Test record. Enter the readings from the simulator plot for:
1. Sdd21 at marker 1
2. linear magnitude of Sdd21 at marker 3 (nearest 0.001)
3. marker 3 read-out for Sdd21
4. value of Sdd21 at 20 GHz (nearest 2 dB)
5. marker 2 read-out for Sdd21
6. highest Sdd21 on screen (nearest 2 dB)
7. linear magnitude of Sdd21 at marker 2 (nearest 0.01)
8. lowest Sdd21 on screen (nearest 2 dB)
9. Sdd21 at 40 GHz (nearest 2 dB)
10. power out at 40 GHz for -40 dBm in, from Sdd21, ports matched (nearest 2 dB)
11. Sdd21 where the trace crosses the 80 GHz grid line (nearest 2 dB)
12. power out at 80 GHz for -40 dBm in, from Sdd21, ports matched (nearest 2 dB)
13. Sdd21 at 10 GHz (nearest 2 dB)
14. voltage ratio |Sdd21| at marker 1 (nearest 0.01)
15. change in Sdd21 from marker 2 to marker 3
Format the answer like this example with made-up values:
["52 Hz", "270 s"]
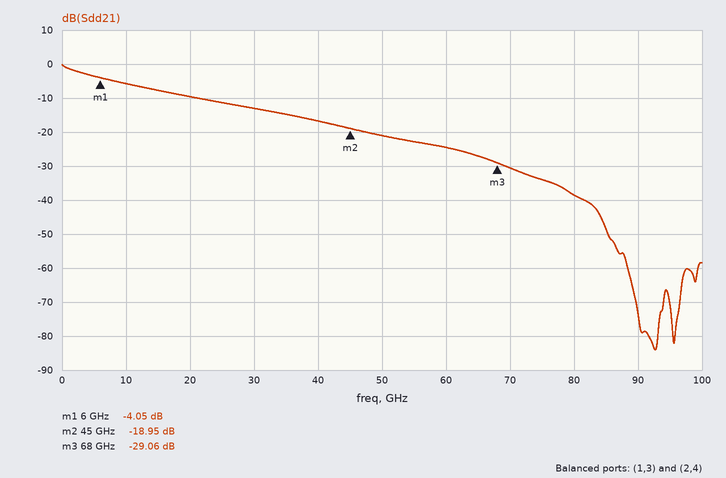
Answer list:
["-4.05 dB", "0.035", "-29.06 dB", "-10 dB", "-18.95 dB", "0 dB", "0.11", "-84 dB", "-16 dB", "-56 dBm", "-38 dB", "-78 dBm", "-6 dB", "0.63", "-10.11 dB"]
